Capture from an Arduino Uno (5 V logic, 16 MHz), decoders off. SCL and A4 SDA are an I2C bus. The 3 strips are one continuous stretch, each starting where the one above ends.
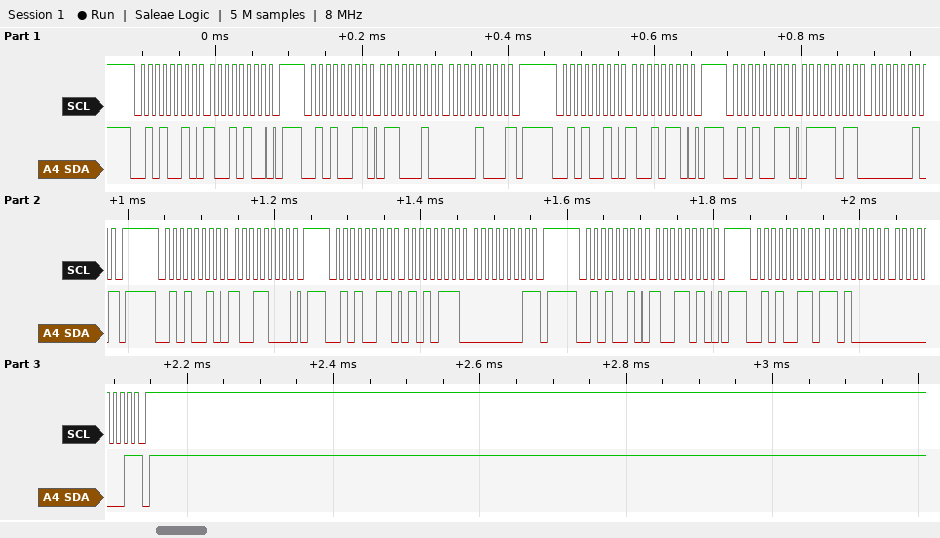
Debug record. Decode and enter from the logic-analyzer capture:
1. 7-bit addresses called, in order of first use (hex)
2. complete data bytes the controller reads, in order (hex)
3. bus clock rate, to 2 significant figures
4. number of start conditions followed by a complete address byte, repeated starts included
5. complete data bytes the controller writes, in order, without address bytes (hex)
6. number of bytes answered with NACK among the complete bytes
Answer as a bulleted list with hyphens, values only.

- 0x29
- 62 08 7B 02 57 01 D0 01
- 100 kHz
- 8
- 94 96 98 9A
- 4
